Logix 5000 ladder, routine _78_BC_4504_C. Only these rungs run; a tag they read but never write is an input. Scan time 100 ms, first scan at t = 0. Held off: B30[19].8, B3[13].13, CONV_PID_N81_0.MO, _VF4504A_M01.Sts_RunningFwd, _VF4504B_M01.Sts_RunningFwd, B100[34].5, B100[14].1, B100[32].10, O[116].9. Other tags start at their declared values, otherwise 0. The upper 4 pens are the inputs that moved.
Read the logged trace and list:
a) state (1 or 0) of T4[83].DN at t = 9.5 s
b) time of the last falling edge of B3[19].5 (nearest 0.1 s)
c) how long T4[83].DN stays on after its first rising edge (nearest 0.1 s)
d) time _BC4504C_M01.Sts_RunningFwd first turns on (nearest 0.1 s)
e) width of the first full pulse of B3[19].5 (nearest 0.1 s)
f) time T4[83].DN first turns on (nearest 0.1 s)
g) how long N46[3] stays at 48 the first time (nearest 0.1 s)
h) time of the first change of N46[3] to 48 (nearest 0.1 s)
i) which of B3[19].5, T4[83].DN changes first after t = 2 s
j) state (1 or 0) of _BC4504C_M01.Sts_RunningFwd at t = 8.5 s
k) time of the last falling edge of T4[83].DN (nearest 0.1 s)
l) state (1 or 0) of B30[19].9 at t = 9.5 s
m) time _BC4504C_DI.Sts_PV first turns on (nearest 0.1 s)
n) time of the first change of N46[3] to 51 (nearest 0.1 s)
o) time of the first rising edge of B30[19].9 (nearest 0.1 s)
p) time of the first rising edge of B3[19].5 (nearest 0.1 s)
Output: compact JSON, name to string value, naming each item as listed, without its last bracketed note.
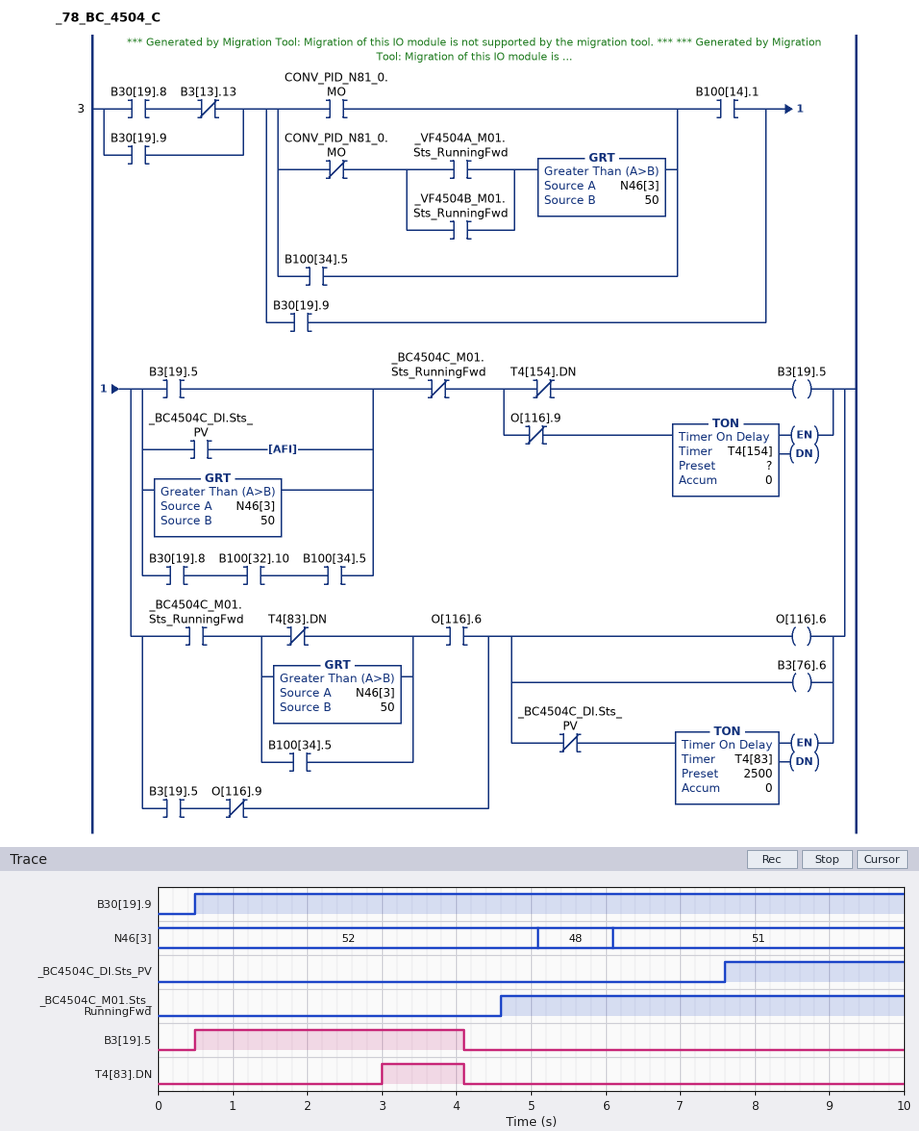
{"state (1 or 0) of T4[83].DN at t = 9.5 s": "0", "time of the last falling edge of B3[19].5": "4.1 s", "how long T4[83].DN stays on after its first rising edge": "1.1 s", "time _BC4504C_M01.Sts_RunningFwd first turns on": "4.6 s", "width of the first full pulse of B3[19].5": "3.6 s", "time T4[83].DN first turns on": "3.0 s", "how long N46[3] stays at 48 the first time": "1.0 s", "time of the first change of N46[3] to 48": "5.1 s", "which of B3[19].5, T4[83].DN changes first after t = 2 s": "T4[83].DN", "state (1 or 0) of _BC4504C_M01.Sts_RunningFwd at t = 8.5 s": "1", "time of the last falling edge of T4[83].DN": "4.1 s", "state (1 or 0) of B30[19].9 at t = 9.5 s": "1", "time _BC4504C_DI.Sts_PV first turns on": "7.6 s", "time of the first change of N46[3] to 51": "6.1 s", "time of the first rising edge of B30[19].9": "0.5 s", "time of the first rising edge of B3[19].5": "0.5 s"}
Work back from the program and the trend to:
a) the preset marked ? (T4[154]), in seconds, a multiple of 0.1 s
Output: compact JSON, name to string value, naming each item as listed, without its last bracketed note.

{"the preset marked ? (T4[154]), in seconds, a multiple of 0.1 s": "3.5 s"}
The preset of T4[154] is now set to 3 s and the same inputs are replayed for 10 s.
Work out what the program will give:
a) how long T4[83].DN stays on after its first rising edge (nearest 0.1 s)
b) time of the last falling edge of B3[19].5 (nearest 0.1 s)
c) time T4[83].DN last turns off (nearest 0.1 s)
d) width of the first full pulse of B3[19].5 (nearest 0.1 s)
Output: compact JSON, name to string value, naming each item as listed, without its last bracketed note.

{"how long T4[83].DN stays on after its first rising edge": "0.6 s", "time of the last falling edge of B3[19].5": "3.6 s", "time T4[83].DN last turns off": "3.6 s", "width of the first full pulse of B3[19].5": "3.1 s"}
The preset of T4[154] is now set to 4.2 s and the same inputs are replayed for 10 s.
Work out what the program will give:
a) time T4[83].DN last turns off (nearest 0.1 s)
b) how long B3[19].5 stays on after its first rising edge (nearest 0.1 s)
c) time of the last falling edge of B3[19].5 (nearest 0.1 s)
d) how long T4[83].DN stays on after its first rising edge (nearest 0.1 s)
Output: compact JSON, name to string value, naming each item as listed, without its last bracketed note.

{"time T4[83].DN last turns off": "5.1 s", "how long B3[19].5 stays on after its first rising edge": "4.1 s", "time of the last falling edge of B3[19].5": "4.6 s", "how long T4[83].DN stays on after its first rising edge": "2.1 s"}
